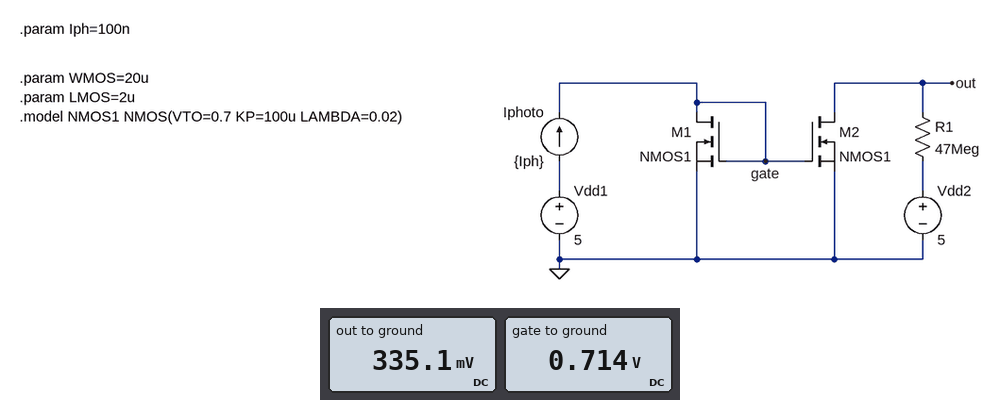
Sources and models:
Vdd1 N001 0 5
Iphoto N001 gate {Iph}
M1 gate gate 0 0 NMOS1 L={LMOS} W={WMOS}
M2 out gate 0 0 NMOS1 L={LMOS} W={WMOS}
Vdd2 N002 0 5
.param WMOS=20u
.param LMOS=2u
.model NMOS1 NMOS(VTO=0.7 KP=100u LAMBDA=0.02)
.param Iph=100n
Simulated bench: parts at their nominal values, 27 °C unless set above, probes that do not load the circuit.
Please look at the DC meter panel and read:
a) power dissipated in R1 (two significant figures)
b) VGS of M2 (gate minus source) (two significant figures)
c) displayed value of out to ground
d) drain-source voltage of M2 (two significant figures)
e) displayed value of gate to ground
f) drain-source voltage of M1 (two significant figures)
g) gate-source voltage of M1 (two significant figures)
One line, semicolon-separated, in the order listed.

460 nW; 710 mV; 335.1 mV; 340 mV; 0.714 V; 710 mV; 710 mV
